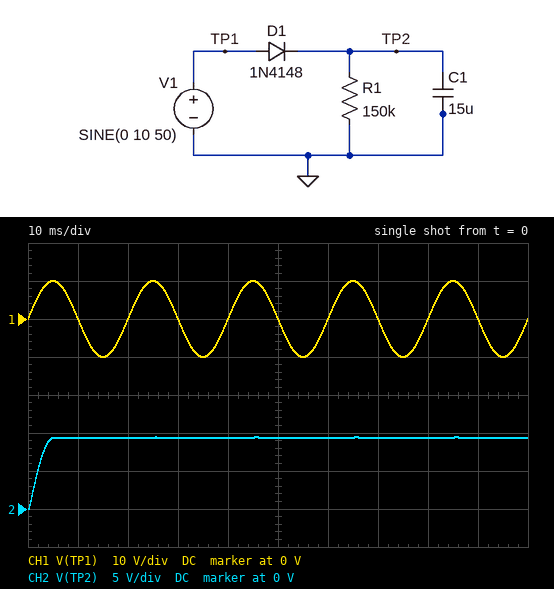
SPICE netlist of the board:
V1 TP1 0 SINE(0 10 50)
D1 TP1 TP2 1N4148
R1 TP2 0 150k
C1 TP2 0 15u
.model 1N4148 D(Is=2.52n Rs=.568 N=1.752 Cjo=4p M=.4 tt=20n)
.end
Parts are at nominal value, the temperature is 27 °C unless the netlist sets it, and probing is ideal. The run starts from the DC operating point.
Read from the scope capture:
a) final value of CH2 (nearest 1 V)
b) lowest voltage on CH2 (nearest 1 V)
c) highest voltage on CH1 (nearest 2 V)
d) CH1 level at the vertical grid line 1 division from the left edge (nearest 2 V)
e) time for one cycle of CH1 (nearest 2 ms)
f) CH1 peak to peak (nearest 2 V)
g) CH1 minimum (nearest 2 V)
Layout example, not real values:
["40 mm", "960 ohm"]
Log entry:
["9 V", "0 V", "10 V", "0 V", "20 ms", "20 V", "-10 V"]
